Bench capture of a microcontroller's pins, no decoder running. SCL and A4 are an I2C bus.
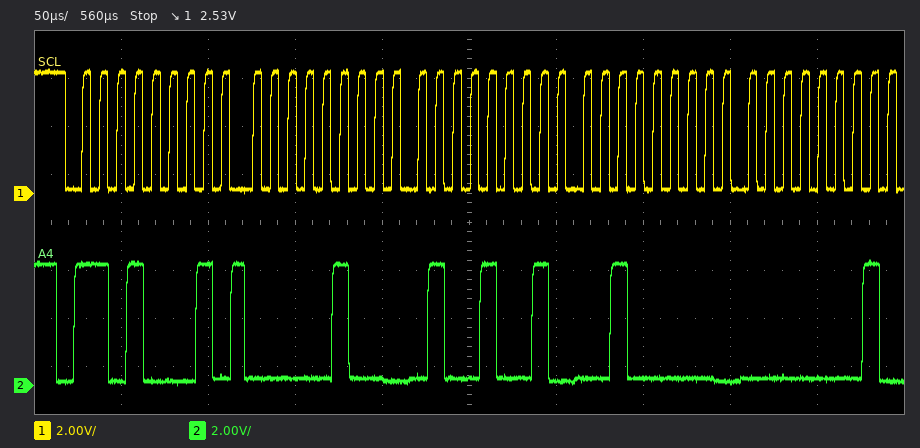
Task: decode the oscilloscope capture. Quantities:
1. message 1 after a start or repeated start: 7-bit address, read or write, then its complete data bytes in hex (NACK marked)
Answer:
0x68 read: 04 49 20 01
